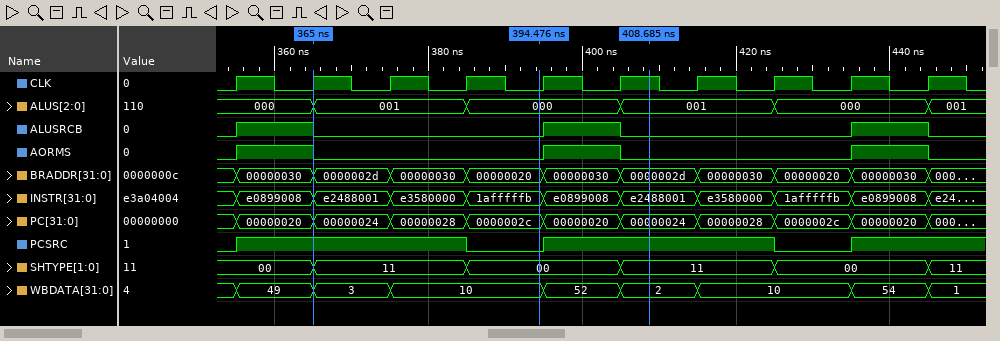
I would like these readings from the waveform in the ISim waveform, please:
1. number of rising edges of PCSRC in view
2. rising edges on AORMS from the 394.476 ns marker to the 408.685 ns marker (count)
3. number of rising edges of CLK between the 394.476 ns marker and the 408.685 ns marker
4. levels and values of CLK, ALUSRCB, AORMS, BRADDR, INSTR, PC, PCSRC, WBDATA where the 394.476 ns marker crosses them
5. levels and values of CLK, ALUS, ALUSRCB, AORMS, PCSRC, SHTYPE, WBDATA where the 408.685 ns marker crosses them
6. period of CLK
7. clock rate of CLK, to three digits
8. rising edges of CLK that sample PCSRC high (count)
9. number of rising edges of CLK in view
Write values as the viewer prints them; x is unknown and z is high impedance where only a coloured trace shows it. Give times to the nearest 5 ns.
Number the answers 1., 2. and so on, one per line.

1. 3
2. 1
3. 2
4. CLK=0, ALUSRCB=0, AORMS=0, BRADDR=00000020, INSTR=1afffffb, PC=0000002c, PCSRC=0, WBDATA=10
5. CLK=1, ALUS=001, ALUSRCB=0, AORMS=0, PCSRC=1, SHTYPE=11, WBDATA=2
6. 10 ns
7. 100 MHz
8. 7
9. 10
